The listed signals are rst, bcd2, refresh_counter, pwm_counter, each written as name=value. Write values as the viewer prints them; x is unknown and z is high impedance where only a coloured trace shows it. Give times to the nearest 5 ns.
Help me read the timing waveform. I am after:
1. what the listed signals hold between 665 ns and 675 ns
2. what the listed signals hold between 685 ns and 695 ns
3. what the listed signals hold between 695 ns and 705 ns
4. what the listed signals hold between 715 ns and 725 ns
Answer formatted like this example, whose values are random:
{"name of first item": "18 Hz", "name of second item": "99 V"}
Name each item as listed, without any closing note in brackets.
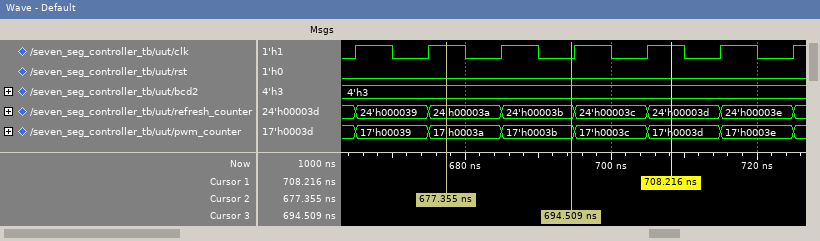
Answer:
{"what the listed signals hold between 665 ns and 675 ns": "rst=0, bcd2=4'h3, refresh_counter=24'h000039, pwm_counter=17'h00039", "what the listed signals hold between 685 ns and 695 ns": "rst=0, bcd2=4'h3, refresh_counter=24'h00003b, pwm_counter=17'h0003b", "what the listed signals hold between 695 ns and 705 ns": "rst=0, bcd2=4'h3, refresh_counter=24'h00003c, pwm_counter=17'h0003c", "what the listed signals hold between 715 ns and 725 ns": "rst=0, bcd2=4'h3, refresh_counter=24'h00003e, pwm_counter=17'h0003e"}
